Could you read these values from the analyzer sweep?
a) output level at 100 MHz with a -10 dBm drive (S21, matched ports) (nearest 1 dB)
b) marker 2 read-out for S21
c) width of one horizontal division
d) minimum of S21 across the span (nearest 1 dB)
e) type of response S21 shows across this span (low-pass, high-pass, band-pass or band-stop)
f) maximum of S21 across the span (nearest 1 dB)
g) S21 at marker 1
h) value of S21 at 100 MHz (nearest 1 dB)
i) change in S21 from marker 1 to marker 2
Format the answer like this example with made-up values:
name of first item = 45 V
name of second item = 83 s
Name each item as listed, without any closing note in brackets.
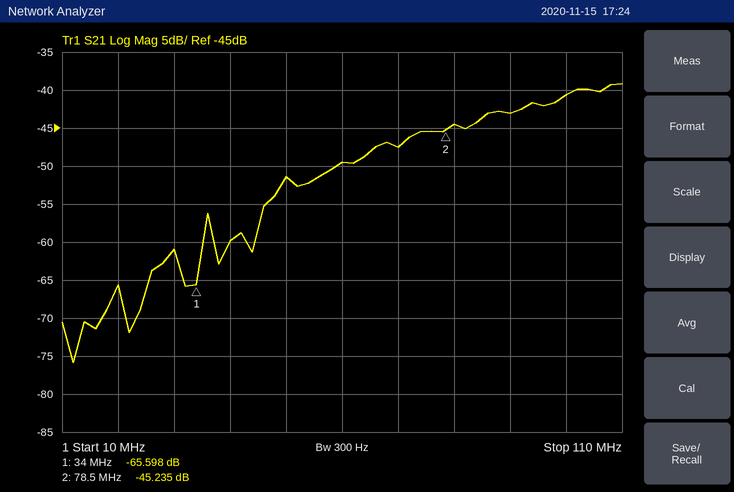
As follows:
output level at 100 MHz with a -10 dBm drive (S21, matched ports) = -51 dBm
marker 2 read-out for S21 = -45.235 dB
width of one horizontal division = 10 MHz
minimum of S21 across the span = -76 dB
type of response S21 shows across this span = high-pass
maximum of S21 across the span = -39 dB
S21 at marker 1 = -65.598 dB
value of S21 at 100 MHz = -41 dB
change in S21 from marker 1 to marker 2 = 20.363 dB
